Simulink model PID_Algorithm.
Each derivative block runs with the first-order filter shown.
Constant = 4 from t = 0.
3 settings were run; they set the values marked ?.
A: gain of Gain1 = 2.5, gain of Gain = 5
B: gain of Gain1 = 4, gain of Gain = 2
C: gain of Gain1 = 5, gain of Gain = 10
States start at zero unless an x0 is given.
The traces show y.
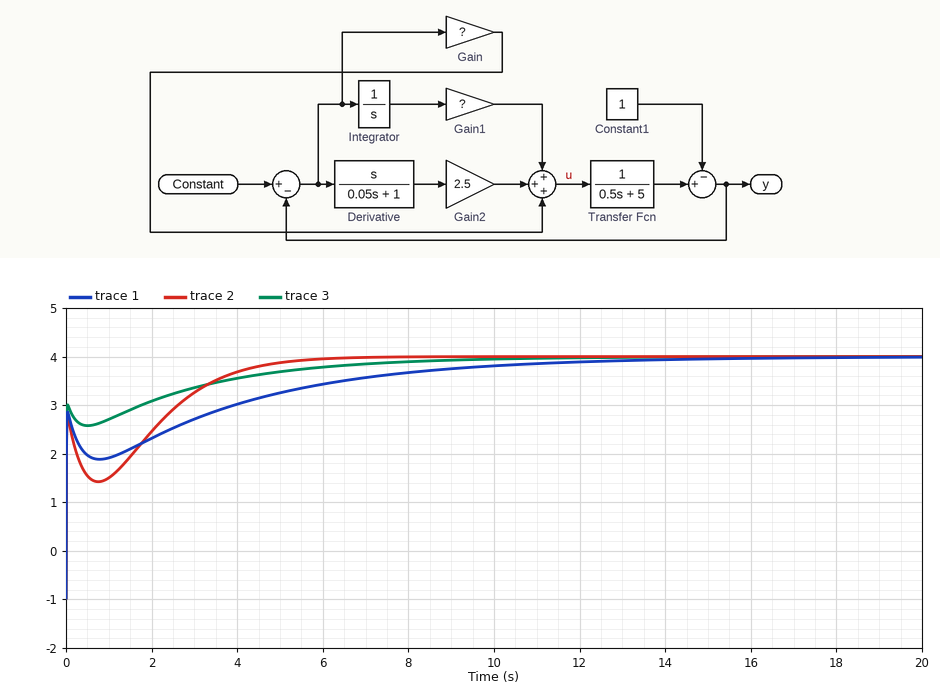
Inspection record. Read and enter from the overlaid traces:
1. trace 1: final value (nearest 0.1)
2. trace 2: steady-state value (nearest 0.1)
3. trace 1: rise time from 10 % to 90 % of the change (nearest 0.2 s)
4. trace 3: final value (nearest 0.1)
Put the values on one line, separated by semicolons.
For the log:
4.0; 4.0; 6.4 s; 4.0
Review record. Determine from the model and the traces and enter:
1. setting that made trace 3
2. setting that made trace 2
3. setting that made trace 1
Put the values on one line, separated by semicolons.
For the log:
C; B; A
